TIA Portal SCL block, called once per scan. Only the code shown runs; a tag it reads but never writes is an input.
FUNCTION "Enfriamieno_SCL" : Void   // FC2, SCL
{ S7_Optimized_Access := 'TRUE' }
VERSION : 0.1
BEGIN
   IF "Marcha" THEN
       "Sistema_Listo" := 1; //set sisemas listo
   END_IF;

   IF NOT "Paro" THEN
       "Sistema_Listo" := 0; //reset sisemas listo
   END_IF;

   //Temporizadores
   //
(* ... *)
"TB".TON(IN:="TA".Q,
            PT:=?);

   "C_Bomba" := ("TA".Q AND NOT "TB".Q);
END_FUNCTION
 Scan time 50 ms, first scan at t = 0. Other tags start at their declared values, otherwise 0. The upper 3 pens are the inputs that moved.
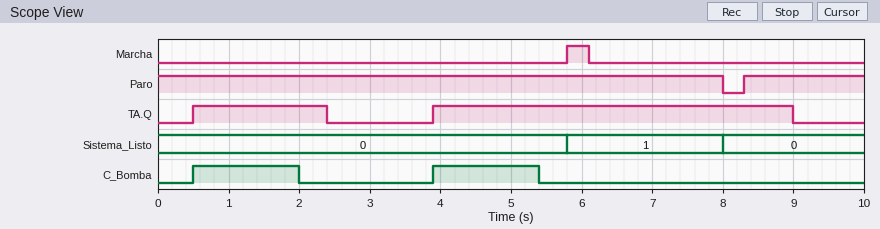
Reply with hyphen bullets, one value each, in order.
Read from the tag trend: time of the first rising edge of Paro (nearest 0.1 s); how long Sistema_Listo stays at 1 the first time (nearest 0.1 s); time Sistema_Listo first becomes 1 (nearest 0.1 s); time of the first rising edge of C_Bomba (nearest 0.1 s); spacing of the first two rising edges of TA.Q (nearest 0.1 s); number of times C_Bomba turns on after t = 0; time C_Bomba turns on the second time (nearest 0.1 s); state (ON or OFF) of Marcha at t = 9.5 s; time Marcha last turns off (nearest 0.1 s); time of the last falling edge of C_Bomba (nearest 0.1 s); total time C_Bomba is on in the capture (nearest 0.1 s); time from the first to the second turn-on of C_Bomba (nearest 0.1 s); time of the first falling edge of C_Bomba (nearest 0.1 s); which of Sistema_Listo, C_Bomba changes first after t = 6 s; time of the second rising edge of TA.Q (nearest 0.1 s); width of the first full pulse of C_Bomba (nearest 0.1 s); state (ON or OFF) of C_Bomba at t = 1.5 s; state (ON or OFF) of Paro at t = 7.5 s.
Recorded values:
- 8.3 s
- 2.2 s
- 5.8 s
- 0.5 s
- 3.4 s
- 2
- 3.9 s
- OFF
- 6.1 s
- 5.4 s
- 3.0 s
- 3.4 s
- 2.0 s
- Sistema_Listo
- 3.9 s
- 1.5 s
- ON
- ON
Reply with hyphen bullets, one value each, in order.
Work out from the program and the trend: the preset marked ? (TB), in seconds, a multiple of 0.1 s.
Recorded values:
- 1.5 s
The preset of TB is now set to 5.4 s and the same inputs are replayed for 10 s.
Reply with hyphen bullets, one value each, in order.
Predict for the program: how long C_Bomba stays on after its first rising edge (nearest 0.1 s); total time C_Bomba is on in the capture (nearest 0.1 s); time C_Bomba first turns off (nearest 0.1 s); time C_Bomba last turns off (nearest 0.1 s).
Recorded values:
- 1.9 s
- 7.0 s
- 2.4 s
- 9.0 s
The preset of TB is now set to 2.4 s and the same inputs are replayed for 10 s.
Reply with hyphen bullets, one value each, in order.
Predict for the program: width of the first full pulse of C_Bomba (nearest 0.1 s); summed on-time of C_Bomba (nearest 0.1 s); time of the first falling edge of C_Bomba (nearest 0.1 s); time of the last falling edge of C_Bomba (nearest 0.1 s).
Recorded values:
- 1.9 s
- 4.3 s
- 2.4 s
- 6.3 s
